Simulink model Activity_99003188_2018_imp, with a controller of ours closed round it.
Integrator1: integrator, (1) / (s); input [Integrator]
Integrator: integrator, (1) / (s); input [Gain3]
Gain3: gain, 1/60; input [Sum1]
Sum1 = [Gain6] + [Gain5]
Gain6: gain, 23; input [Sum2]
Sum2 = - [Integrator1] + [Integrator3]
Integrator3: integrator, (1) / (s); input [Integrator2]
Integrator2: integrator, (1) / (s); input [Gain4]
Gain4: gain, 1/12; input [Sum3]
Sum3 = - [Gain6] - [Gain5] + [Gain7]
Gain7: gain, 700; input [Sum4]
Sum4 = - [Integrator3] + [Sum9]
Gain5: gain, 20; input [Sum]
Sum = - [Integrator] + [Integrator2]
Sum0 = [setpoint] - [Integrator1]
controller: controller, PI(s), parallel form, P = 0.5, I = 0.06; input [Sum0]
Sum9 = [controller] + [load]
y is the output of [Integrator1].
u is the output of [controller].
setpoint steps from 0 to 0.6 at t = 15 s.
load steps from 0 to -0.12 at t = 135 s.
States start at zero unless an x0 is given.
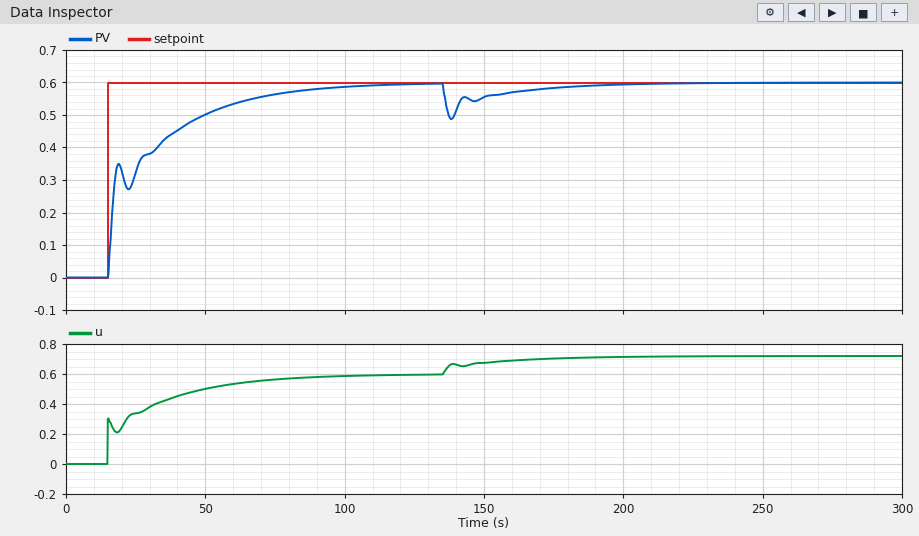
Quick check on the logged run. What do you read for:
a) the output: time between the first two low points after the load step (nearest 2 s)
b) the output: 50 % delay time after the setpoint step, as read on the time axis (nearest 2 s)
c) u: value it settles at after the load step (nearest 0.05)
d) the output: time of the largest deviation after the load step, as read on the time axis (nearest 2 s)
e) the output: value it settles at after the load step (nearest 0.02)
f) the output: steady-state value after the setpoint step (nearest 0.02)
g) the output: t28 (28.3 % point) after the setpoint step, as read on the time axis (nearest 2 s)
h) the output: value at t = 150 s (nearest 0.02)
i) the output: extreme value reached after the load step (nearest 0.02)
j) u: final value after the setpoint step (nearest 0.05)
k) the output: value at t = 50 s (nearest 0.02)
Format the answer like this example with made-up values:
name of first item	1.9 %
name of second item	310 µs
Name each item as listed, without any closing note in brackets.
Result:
the output: time between the first two low points after the load step	8 s
the output: 50 % delay time after the setpoint step, as read on the time axis	18 s
u: value it settles at after the load step	0.70
the output: time of the largest deviation after the load step, as read on the time axis	138 s
the output: value it settles at after the load step	0.60
the output: steady-state value after the setpoint step	0.60
the output: t28 (28.3 % point) after the setpoint step, as read on the time axis	16 s
the output: value at t = 150 s	0.56
the output: extreme value reached after the load step	0.48
u: final value after the setpoint step	0.60
the output: value at t = 50 s	0.50
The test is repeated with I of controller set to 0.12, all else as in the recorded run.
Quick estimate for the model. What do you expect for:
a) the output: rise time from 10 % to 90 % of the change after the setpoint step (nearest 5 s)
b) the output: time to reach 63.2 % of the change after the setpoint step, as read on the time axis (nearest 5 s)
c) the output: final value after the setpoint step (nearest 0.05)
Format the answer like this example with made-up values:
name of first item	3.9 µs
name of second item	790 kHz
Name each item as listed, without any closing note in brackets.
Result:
the output: rise time from 10 % to 90 % of the change after the setpoint step	25 s
the output: time to reach 63.2 % of the change after the setpoint step, as read on the time axis	20 s
the output: final value after the setpoint step	0.60
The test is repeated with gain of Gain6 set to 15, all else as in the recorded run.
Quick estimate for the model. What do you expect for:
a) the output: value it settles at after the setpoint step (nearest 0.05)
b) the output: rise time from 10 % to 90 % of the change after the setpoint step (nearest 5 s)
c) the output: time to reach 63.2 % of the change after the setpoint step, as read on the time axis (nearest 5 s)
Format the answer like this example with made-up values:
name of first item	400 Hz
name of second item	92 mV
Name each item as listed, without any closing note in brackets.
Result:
the output: value it settles at after the setpoint step	0.60
the output: rise time from 10 % to 90 % of the change after the setpoint step	45 s
the output: time to reach 63.2 % of the change after the setpoint step, as read on the time axis	30 s
